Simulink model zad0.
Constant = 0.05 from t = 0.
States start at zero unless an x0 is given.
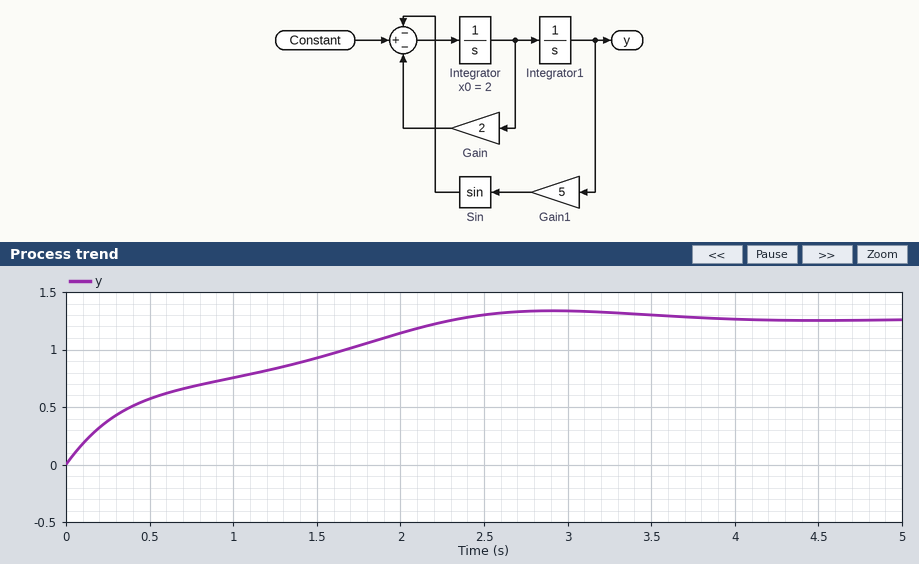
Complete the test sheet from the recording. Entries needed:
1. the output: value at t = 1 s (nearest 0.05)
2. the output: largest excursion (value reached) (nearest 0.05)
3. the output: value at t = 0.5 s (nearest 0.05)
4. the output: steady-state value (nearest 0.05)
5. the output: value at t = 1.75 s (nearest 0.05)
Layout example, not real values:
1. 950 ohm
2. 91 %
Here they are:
1. 0.75
2. 1.35
3. 0.55
4. 1.25
5. 1.05
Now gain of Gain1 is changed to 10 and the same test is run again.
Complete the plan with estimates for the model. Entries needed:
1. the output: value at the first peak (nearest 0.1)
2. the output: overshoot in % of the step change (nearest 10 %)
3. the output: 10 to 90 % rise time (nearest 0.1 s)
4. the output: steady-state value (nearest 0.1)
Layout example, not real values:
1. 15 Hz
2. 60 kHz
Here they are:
1. 0.8
2. 30 %
3. 0.4 s
4. 0.6
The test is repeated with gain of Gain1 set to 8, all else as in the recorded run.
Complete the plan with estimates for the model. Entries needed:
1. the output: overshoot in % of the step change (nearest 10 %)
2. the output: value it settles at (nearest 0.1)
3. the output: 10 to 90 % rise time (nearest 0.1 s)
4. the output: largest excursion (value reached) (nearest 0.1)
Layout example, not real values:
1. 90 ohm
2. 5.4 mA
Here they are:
1. 20 %
2. 0.8
3. 0.6 s
4. 0.9
